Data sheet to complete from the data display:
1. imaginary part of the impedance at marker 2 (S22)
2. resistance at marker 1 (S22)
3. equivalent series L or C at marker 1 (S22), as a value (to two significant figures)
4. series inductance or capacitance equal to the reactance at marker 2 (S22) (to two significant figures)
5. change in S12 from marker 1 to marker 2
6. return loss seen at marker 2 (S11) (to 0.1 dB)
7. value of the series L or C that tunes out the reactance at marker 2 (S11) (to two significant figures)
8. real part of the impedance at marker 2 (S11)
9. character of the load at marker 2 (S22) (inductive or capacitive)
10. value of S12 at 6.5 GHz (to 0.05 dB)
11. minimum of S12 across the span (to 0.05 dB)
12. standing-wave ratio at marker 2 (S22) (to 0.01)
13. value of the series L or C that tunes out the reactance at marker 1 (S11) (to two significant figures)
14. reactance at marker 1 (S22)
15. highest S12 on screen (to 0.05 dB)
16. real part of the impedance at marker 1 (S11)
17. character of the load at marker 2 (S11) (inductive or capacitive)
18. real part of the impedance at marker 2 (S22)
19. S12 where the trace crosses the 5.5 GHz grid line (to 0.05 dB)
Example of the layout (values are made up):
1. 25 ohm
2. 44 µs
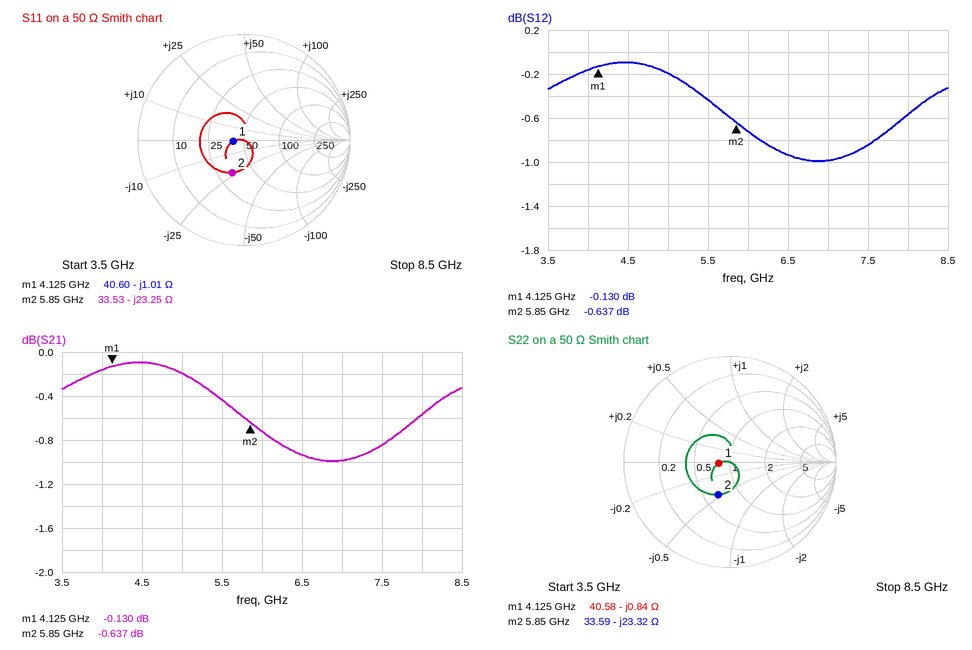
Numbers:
1. -23.32 Ω
2. 40.58 Ω
3. 46 pF
4. 1.2 pF
5. -0.507 dB
6. 9.7 dB
7. 630 pH
8. 33.53 Ω
9. capacitive
10. -0.95 dB
11. -1.00 dB
12. 1.98
13. 39 pH
14. -0.84 Ω
15. -0.10 dB
16. 40.60 Ω
17. capacitive
18. 33.59 Ω
19. -0.45 dB
